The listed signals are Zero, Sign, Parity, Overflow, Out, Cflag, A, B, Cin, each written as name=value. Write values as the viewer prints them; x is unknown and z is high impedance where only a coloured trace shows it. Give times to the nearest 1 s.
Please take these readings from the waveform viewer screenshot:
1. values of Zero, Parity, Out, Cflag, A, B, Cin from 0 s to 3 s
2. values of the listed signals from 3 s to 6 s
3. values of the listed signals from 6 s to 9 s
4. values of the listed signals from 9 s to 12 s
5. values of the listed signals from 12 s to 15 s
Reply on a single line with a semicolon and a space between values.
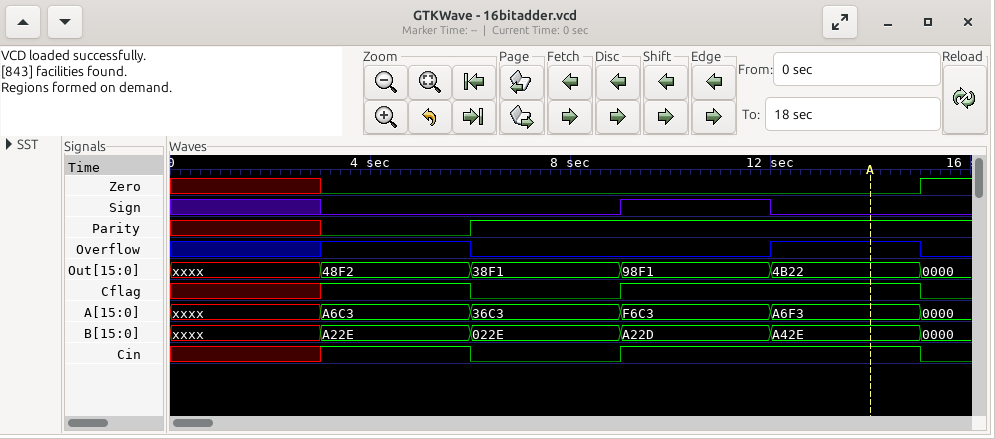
Zero=x, Parity=x, Out=xxxx, Cflag=x, A=xxxx, B=xxxx, Cin=x; Zero=0, Sign=0, Parity=0, Overflow=1, Out=48F2, Cflag=1, A=A6C3, B=A22E, Cin=1; Zero=0, Sign=0, Parity=1, Overflow=0, Out=38F1, Cflag=0, A=36C3, B=022E, Cin=0; Zero=0, Sign=1, Parity=1, Overflow=0, Out=98F1, Cflag=1, A=F6C3, B=A22D, Cin=1; Zero=0, Sign=0, Parity=1, Overflow=1, Out=4B22, Cflag=1, A=A6F3, B=A42E, Cin=1
